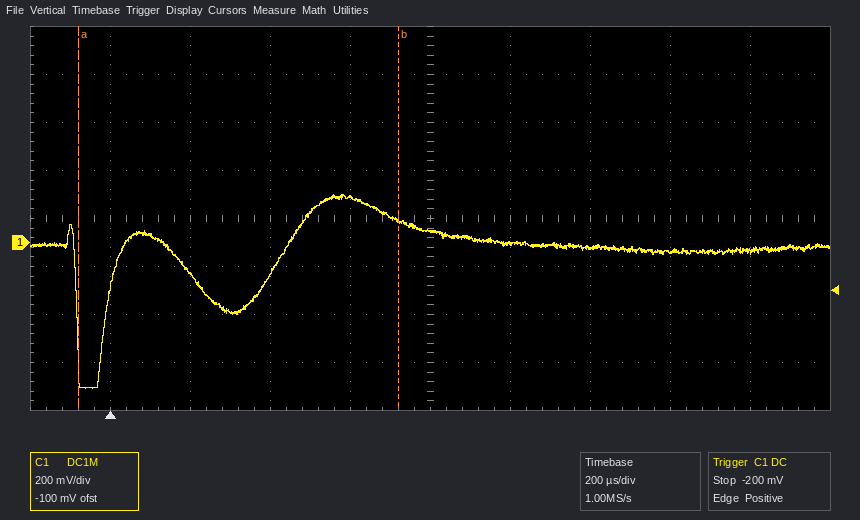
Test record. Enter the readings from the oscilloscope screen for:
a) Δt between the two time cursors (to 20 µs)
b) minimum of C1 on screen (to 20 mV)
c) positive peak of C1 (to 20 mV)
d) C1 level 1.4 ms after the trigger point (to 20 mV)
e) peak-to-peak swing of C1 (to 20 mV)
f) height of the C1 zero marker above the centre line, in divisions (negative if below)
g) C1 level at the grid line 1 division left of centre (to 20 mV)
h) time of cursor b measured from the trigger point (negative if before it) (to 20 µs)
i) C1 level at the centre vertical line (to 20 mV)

800 µs
-600 mV
200 mV
-40 mV
800 mV
-0.5 div
180 mV
+720 µs
40 mV
